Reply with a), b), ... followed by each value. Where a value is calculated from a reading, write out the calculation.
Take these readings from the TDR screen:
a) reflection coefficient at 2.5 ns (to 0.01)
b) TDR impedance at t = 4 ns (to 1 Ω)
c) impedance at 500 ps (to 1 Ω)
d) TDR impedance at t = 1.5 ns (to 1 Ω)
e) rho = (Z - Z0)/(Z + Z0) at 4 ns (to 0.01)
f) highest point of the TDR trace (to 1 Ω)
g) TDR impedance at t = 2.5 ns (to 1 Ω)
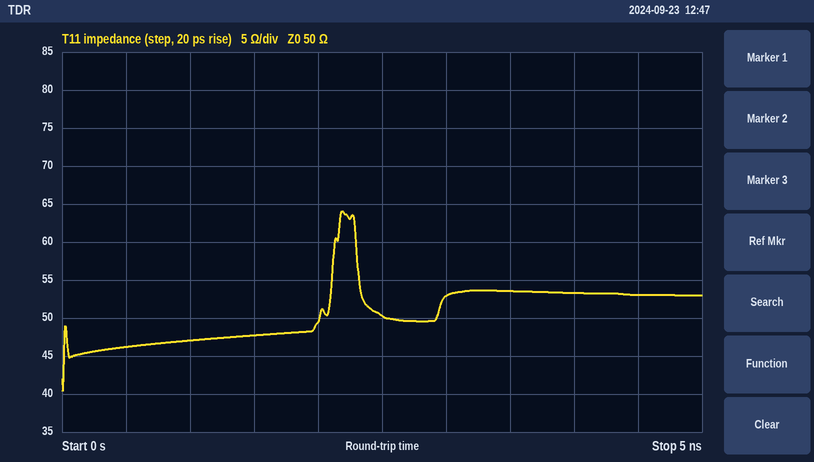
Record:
a) (50 − 50)/(50 + 50) ≈ 0.00
b) 53 Ω
c) 46 Ω
d) 48 Ω
e) (53 − 50)/(53 + 50) ≈ +0.03
f) 64 Ω
g) 50 Ω
